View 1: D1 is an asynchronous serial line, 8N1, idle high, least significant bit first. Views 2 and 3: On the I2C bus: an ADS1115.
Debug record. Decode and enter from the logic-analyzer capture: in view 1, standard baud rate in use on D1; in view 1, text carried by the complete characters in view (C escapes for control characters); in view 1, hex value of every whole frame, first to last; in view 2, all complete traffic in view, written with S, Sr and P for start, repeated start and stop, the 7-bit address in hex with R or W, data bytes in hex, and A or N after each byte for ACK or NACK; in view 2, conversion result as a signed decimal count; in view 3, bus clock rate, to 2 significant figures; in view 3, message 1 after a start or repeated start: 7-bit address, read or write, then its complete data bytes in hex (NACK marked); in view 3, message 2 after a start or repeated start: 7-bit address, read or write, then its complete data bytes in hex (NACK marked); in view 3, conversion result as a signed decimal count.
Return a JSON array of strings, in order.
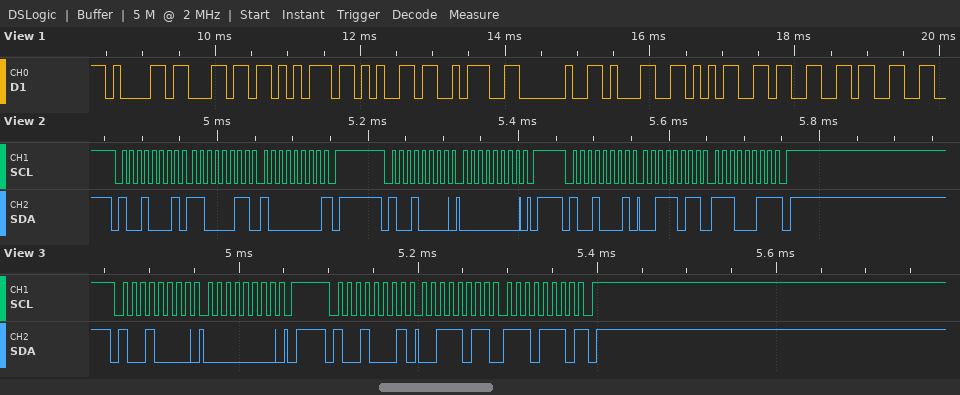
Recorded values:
["9600 baud", "\"alue: 1533\"", "0x61 0x6C 0x75 0x65 0x3A 0x20 0x31 0x35 0x33 0x33", "S 48R A C3 A 80 N P S 48W A 00 A P S 48R A 3B A E3 N P", "15331", "100 kHz", "0x48 write: 00", "0x48 read: 3B EE NACK", "15342"]
